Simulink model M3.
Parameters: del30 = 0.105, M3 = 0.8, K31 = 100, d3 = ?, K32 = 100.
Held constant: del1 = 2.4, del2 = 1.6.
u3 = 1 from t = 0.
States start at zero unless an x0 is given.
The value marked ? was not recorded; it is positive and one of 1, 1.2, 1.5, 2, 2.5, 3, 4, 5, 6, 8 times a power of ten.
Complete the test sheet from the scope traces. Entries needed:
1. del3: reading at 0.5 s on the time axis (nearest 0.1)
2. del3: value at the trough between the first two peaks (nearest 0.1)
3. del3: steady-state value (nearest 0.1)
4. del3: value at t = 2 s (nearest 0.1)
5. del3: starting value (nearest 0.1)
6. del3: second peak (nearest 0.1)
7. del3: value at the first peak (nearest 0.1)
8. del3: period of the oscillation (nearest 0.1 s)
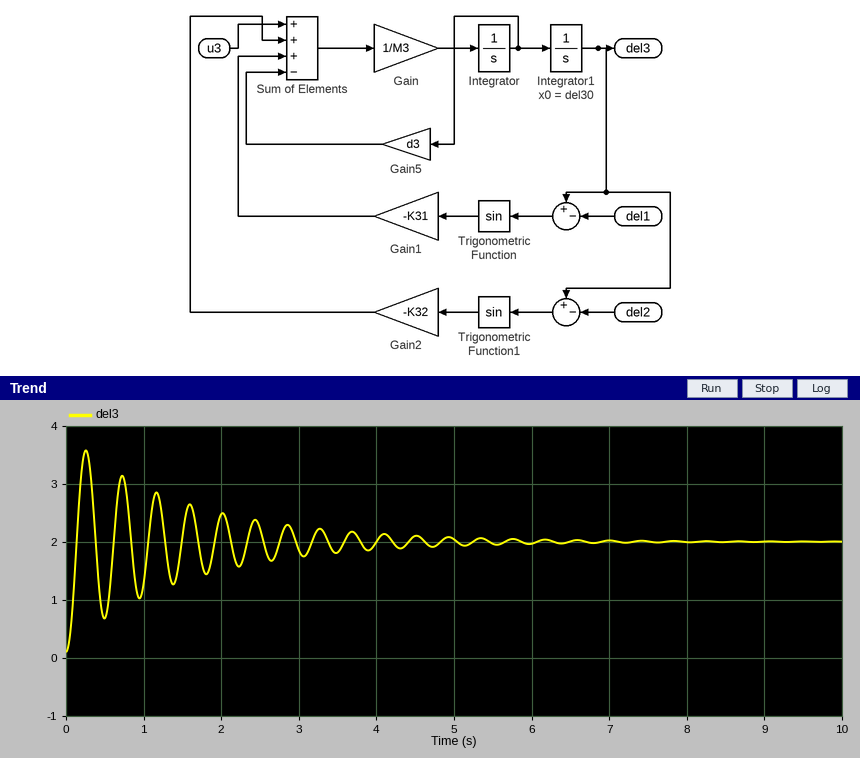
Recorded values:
0.7
0.7
2.0
2.5
0.1
3.1
3.6
0.5 s
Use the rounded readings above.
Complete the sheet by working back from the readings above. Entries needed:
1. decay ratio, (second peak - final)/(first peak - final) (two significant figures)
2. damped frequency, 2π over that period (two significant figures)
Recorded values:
0.69
13 rad/s
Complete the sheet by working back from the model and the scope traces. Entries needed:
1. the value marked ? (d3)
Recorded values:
1
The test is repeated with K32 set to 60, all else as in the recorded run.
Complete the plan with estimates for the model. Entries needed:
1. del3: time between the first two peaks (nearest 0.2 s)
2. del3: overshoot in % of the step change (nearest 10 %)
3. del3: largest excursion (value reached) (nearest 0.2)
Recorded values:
0.6 s
80 %
3.8
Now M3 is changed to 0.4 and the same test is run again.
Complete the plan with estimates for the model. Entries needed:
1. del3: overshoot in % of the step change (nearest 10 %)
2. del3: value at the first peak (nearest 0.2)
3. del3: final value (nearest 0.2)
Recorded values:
80 %
3.4
2.0
